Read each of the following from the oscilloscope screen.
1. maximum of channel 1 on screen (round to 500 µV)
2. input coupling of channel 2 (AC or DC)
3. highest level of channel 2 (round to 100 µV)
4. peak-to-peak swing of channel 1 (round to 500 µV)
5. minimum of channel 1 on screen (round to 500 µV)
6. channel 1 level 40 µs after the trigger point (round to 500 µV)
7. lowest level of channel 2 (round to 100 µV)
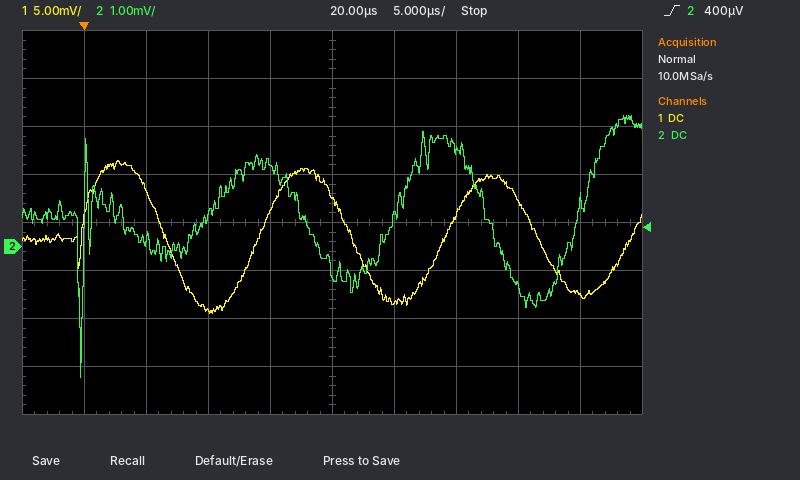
9.0 mV
DC
2.7 mV
16.0 mV
-7.0 mV
-5.0 mV
-2.7 mV
